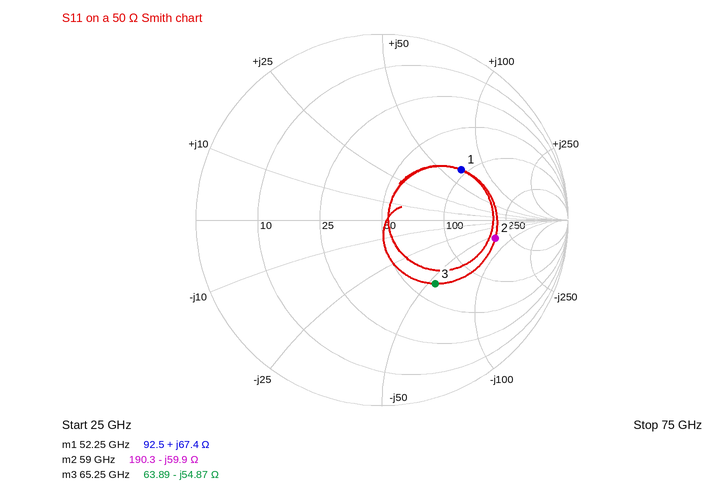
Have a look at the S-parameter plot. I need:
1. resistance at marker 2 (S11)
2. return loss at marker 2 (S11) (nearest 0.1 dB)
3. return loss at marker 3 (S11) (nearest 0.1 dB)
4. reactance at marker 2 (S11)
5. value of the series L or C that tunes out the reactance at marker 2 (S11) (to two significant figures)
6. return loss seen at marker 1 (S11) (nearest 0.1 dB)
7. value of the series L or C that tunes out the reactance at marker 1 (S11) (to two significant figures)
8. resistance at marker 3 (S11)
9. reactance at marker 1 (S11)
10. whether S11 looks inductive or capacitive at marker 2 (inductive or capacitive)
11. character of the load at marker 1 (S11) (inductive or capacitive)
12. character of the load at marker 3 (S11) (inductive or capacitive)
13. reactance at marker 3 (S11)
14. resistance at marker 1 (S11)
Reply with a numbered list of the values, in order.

1. 190.3 Ω
2. 4.2 dB
3. 7.0 dB
4. -59.9 Ω
5. 160 pH
6. 5.9 dB
7. 45 fF
8. 63.89 Ω
9. +67.4 Ω
10. capacitive
11. inductive
12. capacitive
13. -54.87 Ω
14. 92.5 Ω
